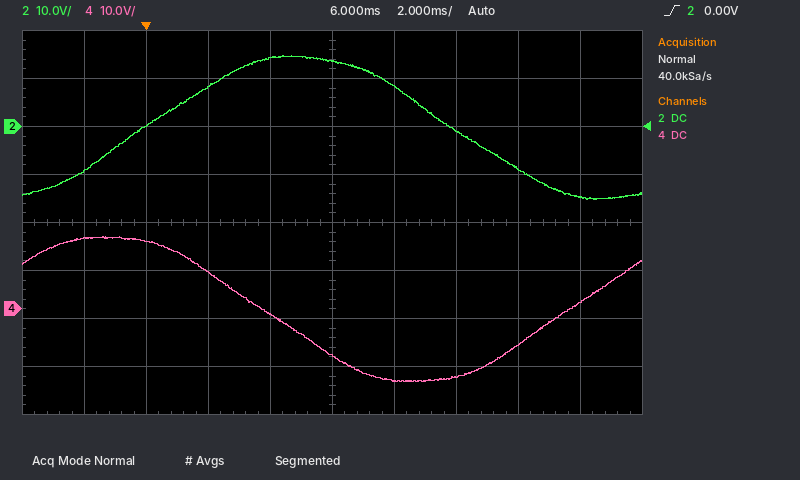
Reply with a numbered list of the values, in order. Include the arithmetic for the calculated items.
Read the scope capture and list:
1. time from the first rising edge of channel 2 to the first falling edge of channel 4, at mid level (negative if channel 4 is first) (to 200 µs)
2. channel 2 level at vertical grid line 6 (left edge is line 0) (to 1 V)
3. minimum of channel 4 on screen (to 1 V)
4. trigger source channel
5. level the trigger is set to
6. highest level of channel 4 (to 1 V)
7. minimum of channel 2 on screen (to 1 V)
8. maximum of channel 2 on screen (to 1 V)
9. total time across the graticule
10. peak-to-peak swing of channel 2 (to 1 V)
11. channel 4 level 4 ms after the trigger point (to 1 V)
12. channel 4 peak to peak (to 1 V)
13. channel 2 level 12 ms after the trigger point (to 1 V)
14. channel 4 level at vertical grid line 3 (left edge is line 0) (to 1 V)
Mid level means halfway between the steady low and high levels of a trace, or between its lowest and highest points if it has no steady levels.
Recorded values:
1. +3.8 ms
2. 8 V
3. -15 V
4. channel 2
5. 0.00 V
6. 15 V
7. -15 V
8. 15 V
9. 20 ms
10. 15 V − (-15 V) = 30 V
11. -1 V
12. 15 V − (-15 V) = 30 V
13. -9 V
14. 8 V
